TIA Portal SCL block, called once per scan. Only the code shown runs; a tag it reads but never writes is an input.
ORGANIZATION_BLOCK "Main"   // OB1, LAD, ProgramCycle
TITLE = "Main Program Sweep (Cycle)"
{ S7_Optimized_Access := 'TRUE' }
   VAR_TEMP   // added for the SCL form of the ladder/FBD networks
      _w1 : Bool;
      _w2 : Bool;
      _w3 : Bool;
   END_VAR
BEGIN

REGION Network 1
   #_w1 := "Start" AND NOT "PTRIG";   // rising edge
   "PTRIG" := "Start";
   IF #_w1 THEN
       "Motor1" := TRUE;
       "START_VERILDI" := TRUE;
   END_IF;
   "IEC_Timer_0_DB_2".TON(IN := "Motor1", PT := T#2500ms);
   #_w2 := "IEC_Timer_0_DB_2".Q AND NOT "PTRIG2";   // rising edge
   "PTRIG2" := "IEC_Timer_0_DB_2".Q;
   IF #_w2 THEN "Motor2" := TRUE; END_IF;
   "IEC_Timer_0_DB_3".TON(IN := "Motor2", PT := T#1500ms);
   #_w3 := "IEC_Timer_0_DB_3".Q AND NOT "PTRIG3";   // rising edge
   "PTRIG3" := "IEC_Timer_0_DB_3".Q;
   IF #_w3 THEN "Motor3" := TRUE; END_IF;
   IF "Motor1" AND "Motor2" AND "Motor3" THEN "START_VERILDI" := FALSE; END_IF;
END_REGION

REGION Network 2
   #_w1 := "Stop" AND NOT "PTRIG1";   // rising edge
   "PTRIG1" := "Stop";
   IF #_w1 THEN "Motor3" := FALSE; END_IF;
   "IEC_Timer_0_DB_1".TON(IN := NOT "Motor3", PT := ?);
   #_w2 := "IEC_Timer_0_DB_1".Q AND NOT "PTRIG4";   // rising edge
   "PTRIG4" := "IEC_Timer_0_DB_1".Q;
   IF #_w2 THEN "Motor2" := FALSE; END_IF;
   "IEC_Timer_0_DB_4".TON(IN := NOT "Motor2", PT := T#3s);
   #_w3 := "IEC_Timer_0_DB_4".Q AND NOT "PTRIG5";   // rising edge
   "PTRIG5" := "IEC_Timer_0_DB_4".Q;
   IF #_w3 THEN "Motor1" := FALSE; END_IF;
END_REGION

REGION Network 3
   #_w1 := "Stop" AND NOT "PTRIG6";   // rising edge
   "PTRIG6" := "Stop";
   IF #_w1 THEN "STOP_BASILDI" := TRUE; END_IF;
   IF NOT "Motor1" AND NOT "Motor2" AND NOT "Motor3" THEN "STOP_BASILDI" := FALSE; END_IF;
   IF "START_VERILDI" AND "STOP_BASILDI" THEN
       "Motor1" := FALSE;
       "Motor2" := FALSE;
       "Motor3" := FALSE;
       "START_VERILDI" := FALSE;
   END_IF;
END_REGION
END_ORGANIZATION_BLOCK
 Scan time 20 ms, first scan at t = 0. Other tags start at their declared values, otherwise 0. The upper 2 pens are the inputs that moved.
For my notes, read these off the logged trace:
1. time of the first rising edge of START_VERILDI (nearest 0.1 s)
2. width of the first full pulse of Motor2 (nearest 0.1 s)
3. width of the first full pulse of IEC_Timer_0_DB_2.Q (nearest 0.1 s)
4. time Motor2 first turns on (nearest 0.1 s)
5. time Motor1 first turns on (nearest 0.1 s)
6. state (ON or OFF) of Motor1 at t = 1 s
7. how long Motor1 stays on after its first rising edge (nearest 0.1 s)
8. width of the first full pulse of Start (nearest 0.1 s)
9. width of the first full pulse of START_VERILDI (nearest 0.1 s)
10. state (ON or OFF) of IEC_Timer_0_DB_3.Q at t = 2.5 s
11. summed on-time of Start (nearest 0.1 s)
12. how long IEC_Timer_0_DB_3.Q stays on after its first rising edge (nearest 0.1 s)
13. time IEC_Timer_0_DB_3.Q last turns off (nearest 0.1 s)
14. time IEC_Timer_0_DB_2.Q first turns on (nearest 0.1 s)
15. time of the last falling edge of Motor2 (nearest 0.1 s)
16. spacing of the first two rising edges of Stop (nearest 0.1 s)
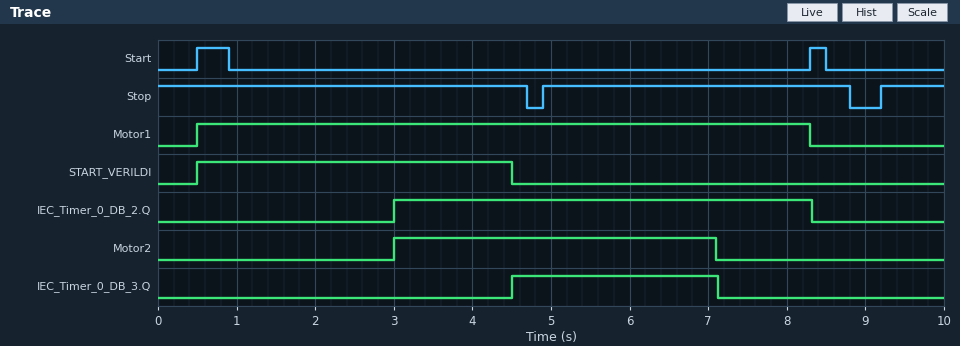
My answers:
0.5 s
4.1 s
5.3 s
3.0 s
0.5 s
ON
7.8 s
0.4 s
4.0 s
OFF
0.6 s
2.6 s
7.1 s
3.0 s
7.1 s
4.3 s
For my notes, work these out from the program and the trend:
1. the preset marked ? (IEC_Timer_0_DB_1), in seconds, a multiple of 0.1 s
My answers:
2.2 s
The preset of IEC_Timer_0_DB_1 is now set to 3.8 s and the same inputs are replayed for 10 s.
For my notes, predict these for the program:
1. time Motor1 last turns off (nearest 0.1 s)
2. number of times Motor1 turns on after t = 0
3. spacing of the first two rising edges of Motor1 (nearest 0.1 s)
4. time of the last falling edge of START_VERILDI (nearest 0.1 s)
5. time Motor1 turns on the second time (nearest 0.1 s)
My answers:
9.2 s
2
7.8 s
9.2 s
8.3 s
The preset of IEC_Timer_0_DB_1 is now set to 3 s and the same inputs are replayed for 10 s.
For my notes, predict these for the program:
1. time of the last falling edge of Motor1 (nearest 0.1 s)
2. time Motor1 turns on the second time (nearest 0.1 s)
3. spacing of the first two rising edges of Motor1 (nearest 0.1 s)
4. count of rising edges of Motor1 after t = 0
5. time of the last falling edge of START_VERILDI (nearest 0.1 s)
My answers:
9.2 s
8.3 s
7.8 s
2
9.2 s
